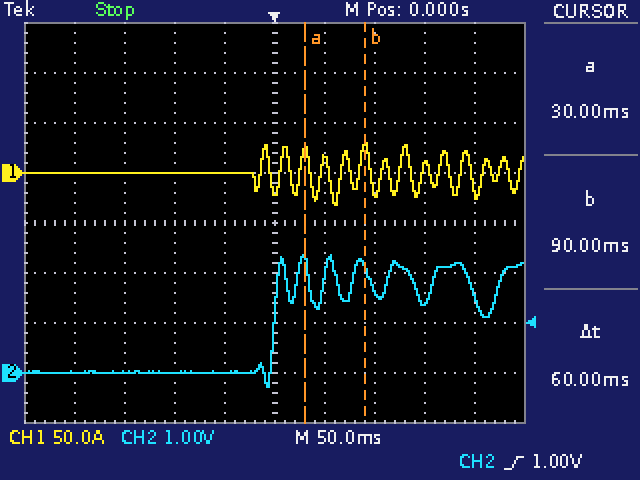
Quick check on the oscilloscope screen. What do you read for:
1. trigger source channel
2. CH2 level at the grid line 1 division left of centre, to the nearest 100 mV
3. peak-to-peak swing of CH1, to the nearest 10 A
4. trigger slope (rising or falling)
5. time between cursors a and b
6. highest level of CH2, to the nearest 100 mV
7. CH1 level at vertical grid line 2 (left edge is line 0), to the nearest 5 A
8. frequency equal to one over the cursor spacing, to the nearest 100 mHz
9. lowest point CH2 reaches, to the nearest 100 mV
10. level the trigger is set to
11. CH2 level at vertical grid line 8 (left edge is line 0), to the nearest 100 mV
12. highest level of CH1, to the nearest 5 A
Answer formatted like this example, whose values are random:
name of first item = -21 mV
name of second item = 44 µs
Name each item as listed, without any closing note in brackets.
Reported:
trigger source channel = CH2
CH2 level at the grid line 1 division left of centre, to the nearest 100 mV = 0.0 V
peak-to-peak swing of CH1, to the nearest 10 A = 60 A
trigger slope = rising
time between cursors a and b = 60 ms
highest level of CH2, to the nearest 100 mV = 2.4 V
CH1 level at vertical grid line 2 (left edge is line 0), to the nearest 5 A = 0 A
frequency equal to one over the cursor spacing, to the nearest 100 mHz = 16.7 Hz
lowest point CH2 reaches, to the nearest 100 mV = -300 mV
level the trigger is set to = 1.00 V
CH2 level at vertical grid line 8 (left edge is line 0), to the nearest 100 mV = 1.4 V
highest level of CH1, to the nearest 5 A = 30 A
